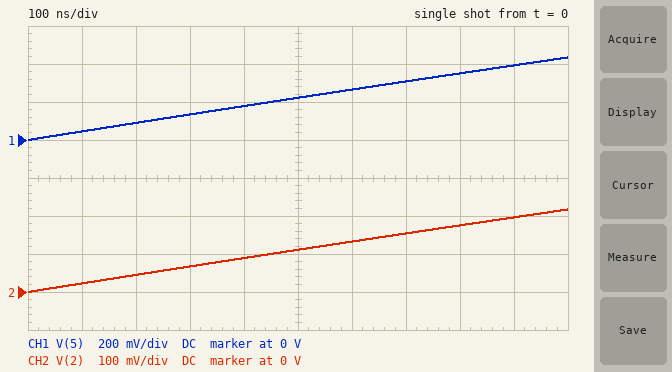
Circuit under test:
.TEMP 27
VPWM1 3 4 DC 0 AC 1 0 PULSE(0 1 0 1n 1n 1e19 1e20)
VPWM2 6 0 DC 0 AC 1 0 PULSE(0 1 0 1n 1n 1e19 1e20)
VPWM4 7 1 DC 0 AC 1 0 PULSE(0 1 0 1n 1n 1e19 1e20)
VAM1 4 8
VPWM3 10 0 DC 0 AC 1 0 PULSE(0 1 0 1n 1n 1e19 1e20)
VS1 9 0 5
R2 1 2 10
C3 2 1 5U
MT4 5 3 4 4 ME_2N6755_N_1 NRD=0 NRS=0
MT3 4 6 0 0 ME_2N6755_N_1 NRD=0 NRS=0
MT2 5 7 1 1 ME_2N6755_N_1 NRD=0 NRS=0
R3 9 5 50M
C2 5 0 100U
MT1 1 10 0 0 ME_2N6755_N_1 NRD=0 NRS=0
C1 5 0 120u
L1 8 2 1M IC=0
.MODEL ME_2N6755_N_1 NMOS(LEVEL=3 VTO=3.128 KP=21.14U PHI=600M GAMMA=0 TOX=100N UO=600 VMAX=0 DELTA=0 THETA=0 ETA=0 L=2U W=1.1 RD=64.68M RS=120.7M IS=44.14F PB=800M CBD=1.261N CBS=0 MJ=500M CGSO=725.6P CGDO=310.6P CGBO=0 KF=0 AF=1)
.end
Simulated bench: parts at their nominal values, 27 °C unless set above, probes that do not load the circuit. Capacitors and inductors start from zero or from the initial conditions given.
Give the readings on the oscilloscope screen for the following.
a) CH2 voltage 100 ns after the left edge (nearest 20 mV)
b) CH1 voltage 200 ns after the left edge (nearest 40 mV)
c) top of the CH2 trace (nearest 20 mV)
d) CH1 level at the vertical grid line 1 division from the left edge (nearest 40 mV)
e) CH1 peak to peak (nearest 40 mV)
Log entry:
20 mV
80 mV
220 mV
40 mV
440 mV
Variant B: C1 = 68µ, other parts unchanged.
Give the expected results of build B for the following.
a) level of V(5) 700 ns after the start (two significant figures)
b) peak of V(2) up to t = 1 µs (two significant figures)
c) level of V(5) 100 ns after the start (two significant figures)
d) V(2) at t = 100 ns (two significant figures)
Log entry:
400 mV
280 mV
59 mV
30 mV
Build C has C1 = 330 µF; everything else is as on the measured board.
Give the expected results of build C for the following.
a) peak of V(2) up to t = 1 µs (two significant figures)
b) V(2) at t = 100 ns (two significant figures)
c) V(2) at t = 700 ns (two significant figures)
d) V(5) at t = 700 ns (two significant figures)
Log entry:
110 mV
12 mV
80 mV
160 mV
